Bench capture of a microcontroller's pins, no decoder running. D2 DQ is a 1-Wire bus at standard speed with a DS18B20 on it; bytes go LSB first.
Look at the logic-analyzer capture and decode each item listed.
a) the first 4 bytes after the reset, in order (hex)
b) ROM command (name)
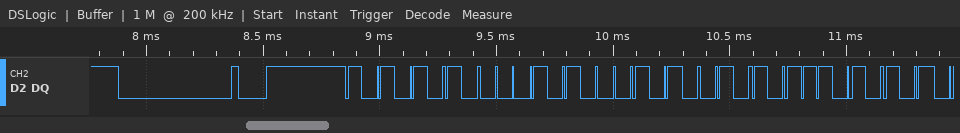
55 28 4A 5D
Match ROM
